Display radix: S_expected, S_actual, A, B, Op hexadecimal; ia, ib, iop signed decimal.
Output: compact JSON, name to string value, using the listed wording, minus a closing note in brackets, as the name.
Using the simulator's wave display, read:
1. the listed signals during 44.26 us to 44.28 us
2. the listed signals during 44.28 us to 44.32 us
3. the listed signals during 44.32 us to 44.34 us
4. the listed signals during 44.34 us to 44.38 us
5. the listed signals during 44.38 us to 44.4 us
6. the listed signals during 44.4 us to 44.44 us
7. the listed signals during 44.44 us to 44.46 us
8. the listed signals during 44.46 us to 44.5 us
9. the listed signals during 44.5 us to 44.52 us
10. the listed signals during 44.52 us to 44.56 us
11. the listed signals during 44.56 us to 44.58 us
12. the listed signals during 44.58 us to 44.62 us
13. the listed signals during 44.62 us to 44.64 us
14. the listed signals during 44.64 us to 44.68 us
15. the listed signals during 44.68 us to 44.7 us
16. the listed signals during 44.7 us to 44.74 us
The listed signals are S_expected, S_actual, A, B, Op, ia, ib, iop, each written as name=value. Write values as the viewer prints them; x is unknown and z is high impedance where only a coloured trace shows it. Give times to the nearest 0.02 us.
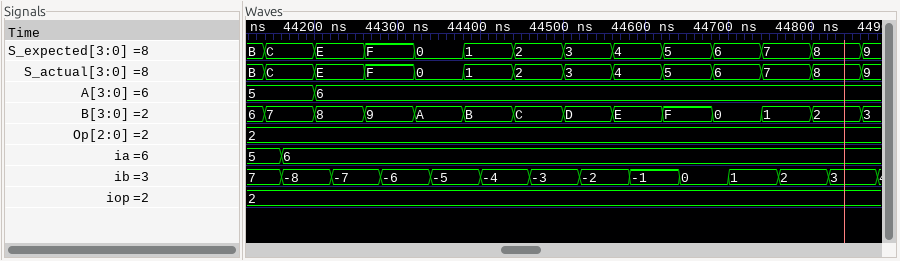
{"the listed signals during 44.26 us to 44.28 us": "S_expected=F, S_actual=F, A=6, B=9, Op=2, ia=6, ib=-7, iop=2", "the listed signals during 44.28 us to 44.32 us": "S_expected=F, S_actual=F, A=6, B=9, Op=2, ia=6, ib=-6, iop=2", "the listed signals during 44.32 us to 44.34 us": "S_expected=0, S_actual=0, A=6, B=A, Op=2, ia=6, ib=-6, iop=2", "the listed signals during 44.34 us to 44.38 us": "S_expected=0, S_actual=0, A=6, B=A, Op=2, ia=6, ib=-5, iop=2", "the listed signals during 44.38 us to 44.4 us": "S_expected=1, S_actual=1, A=6, B=B, Op=2, ia=6, ib=-5, iop=2", "the listed signals during 44.4 us to 44.44 us": "S_expected=1, S_actual=1, A=6, B=B, Op=2, ia=6, ib=-4, iop=2", "the listed signals during 44.44 us to 44.46 us": "S_expected=2, S_actual=2, A=6, B=C, Op=2, ia=6, ib=-4, iop=2", "the listed signals during 44.46 us to 44.5 us": "S_expected=2, S_actual=2, A=6, B=C, Op=2, ia=6, ib=-3, iop=2", "the listed signals during 44.5 us to 44.52 us": "S_expected=3, S_actual=3, A=6, B=D, Op=2, ia=6, ib=-3, iop=2", "the listed signals during 44.52 us to 44.56 us": "S_expected=3, S_actual=3, A=6, B=D, Op=2, ia=6, ib=-2, iop=2", "the listed signals during 44.56 us to 44.58 us": "S_expected=4, S_actual=4, A=6, B=E, Op=2, ia=6, ib=-2, iop=2", "the listed signals during 44.58 us to 44.62 us": "S_expected=4, S_actual=4, A=6, B=E, Op=2, ia=6, ib=-1, iop=2", "the listed signals during 44.62 us to 44.64 us": "S_expected=5, S_actual=5, A=6, B=F, Op=2, ia=6, ib=-1, iop=2", "the listed signals during 44.64 us to 44.68 us": "S_expected=5, S_actual=5, A=6, B=F, Op=2, ia=6, ib=0, iop=2", "the listed signals during 44.68 us to 44.7 us": "S_expected=6, S_actual=6, A=6, B=0, Op=2, ia=6, ib=0, iop=2", "the listed signals during 44.7 us to 44.74 us": "S_expected=6, S_actual=6, A=6, B=0, Op=2, ia=6, ib=1, iop=2"}
